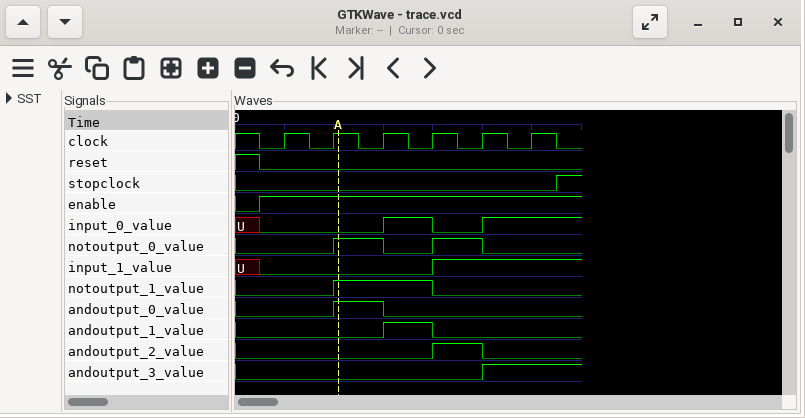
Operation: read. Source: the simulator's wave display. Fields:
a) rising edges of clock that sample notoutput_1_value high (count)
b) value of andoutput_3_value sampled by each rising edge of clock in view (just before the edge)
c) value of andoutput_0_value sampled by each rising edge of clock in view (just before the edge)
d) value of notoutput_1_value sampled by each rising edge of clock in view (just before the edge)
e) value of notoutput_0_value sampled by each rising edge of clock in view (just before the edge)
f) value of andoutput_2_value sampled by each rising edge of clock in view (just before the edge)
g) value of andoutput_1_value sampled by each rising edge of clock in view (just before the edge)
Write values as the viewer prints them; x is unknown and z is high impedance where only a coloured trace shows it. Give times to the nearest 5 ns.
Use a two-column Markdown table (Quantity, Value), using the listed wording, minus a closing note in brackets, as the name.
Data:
| Quantity | Value |
|---|---|
| rising edges of clock that sample notoutput_1_value high | 2 |
| value of andoutput_3_value sampled by each rising edge of clock in view | 0 0 0 0 0 1 |
| value of andoutput_0_value sampled by each rising edge of clock in view | 0 0 1 0 0 0 |
| value of notoutput_1_value sampled by each rising edge of clock in view | 0 0 1 1 0 0 |
| value of notoutput_0_value sampled by each rising edge of clock in view | 0 0 1 0 1 0 |
| value of andoutput_2_value sampled by each rising edge of clock in view | 0 0 0 0 1 0 |
| value of andoutput_1_value sampled by each rising edge of clock in view | 0 0 0 1 0 0 |
